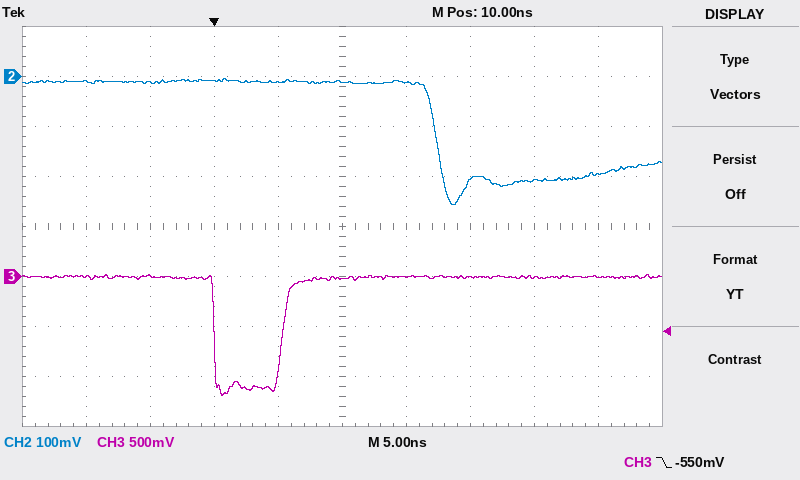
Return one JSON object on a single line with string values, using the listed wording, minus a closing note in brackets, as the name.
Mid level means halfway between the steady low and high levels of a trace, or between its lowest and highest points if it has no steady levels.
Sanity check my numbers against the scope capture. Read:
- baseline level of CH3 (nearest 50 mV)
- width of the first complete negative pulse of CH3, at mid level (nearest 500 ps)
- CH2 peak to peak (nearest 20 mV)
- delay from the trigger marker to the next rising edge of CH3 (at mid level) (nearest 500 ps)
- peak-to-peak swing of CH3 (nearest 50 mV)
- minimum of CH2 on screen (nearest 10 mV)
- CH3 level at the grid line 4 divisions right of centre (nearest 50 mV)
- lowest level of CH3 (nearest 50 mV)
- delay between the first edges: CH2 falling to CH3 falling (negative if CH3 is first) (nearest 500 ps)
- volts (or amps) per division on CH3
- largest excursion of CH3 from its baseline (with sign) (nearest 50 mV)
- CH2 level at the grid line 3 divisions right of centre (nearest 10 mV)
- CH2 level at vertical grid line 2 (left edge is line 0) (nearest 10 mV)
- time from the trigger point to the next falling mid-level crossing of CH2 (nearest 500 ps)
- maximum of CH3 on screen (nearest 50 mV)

{"baseline level of CH3": "0 mV", "width of the first complete negative pulse of CH3, at mid level": "5.5 ns", "CH2 peak to peak": "260 mV", "delay from the trigger marker to the next rising edge of CH3 (at mid level)": "5.5 ns", "peak-to-peak swing of CH3": "1.20 V", "minimum of CH2 on screen": "-260 mV", "CH3 level at the grid line 4 divisions right of centre": "0 mV", "lowest level of CH3": "-1.20 V", "delay between the first edges: CH2 falling to CH3 falling (negative if CH3 is first)": "-17.5 ns", "volts (or amps) per division on CH3": "500 mV", "largest excursion of CH3 from its baseline (with sign)": "-1.20 V", "CH2 level at the grid line 3 divisions right of centre": "-210 mV", "CH2 level at vertical grid line 2 (left edge is line 0)": "-10 mV", "time from the trigger point to the next falling mid-level crossing of CH2": "17.5 ns", "maximum of CH3 on screen": "0 mV"}
